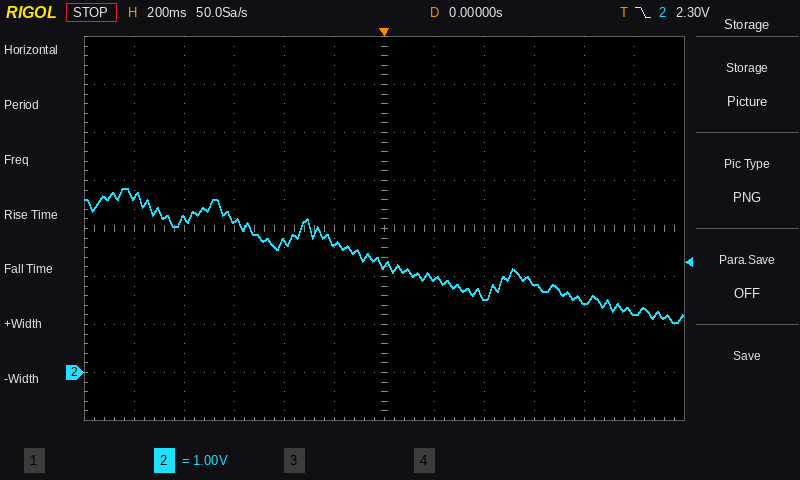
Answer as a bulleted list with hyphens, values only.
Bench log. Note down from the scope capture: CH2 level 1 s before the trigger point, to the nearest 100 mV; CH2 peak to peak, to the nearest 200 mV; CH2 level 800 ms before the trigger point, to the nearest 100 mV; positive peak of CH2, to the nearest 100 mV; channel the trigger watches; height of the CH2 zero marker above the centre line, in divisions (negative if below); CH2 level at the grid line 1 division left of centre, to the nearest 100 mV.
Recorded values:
- 3.7 V
- 2.8 V
- 3.2 V
- 3.8 V
- CH2
- -3.0 div
- 2.7 V
